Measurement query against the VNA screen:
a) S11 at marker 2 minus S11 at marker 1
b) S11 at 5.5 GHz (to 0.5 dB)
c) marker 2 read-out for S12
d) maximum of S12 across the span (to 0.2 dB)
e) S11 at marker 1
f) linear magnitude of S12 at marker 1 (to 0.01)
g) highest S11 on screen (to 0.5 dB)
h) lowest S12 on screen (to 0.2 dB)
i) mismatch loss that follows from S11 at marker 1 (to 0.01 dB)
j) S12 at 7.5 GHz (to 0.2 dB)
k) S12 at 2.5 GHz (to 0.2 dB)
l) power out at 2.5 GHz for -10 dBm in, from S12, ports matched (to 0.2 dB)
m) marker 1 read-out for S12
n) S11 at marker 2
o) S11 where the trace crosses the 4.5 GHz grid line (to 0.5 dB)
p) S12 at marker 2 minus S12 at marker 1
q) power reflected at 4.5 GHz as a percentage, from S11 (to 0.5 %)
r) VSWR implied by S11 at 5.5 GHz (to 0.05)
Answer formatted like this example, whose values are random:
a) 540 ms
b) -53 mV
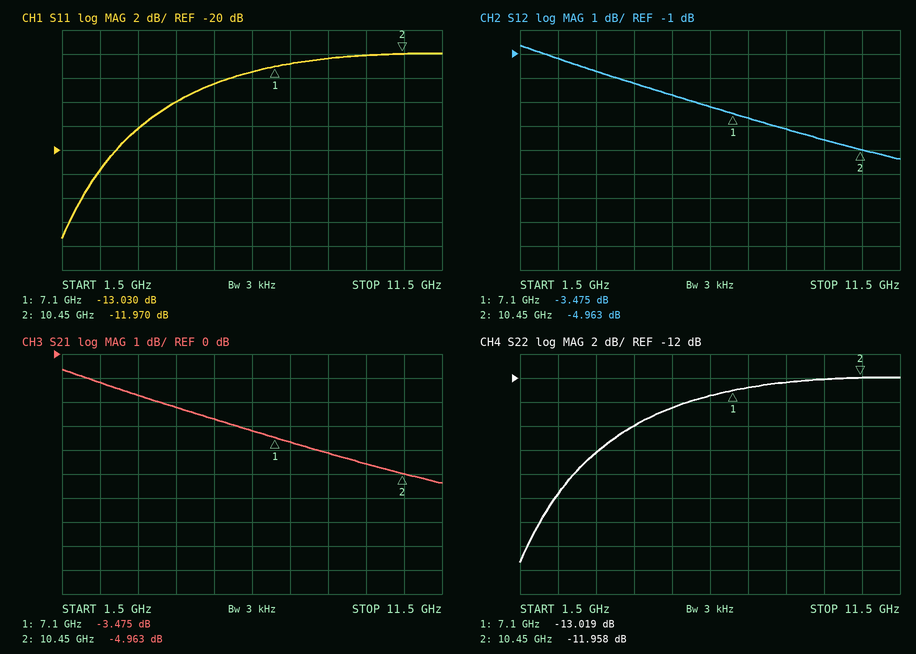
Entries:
a) 1.060 dB
b) -14.5 dB
c) -4.963 dB
d) -0.6 dB
e) -13.030 dB
f) 0.67
g) -12.0 dB
h) -5.4 dB
i) 0.22 dB
j) -3.6 dB
k) -1.2 dB
l) -11.2 dBm
m) -3.475 dB
n) -11.970 dB
o) -16.0 dB
p) -1.488 dB
q) 2.5 %
r) 1.45
